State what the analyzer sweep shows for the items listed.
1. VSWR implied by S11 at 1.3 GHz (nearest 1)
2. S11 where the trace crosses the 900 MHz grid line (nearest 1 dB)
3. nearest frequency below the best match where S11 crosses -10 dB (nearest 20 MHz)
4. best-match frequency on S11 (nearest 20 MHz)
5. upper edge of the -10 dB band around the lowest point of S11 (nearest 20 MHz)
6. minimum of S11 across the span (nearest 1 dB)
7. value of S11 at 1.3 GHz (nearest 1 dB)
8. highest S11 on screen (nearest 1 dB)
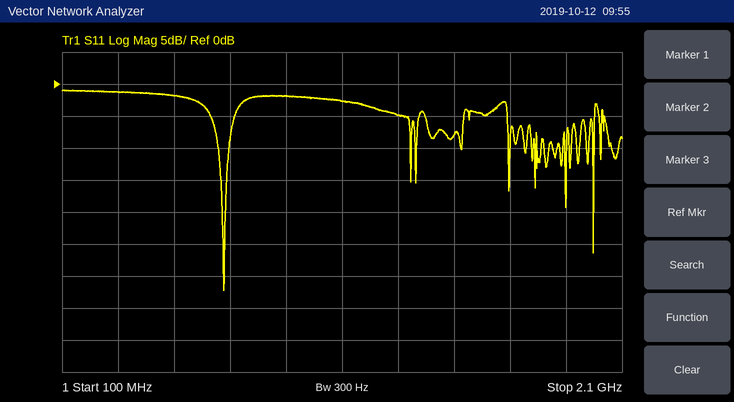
4
-2 dB
660 MHz
680 MHz
700 MHz
-32 dB
-5 dB
-1 dB
